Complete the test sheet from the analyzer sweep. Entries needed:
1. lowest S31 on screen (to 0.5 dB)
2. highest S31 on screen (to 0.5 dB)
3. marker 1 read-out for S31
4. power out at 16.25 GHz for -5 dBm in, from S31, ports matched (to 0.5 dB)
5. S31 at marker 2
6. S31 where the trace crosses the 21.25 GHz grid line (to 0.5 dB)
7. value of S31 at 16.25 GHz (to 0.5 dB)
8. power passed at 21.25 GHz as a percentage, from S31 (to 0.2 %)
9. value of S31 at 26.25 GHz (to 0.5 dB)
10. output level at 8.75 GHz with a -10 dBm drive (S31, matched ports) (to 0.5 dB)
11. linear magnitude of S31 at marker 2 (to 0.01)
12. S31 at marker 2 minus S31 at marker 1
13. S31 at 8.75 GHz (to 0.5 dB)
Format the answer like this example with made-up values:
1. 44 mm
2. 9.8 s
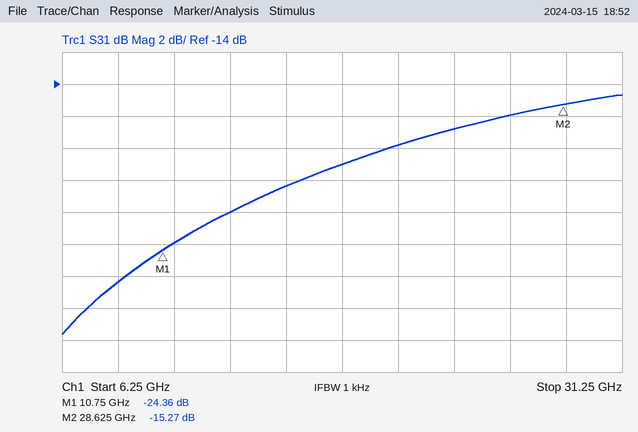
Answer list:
1. -29.5 dB
2. -14.5 dB
3. -24.36 dB
4. -25.5 dBm
5. -15.27 dB
6. -18.0 dB
7. -20.5 dB
8. 1.6 %
9. -16.0 dB
10. -36.5 dBm
11. 0.17
12. 9.09 dB
13. -26.5 dB
